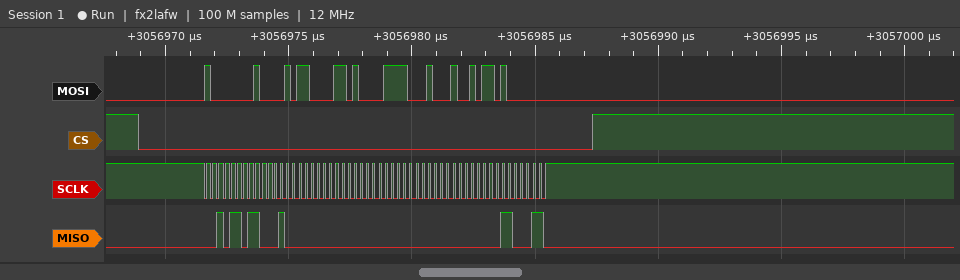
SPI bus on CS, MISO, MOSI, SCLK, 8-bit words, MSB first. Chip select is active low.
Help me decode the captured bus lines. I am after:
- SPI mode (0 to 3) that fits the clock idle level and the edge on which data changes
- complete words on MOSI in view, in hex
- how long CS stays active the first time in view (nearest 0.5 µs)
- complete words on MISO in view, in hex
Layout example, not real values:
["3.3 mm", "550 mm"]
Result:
["3", "80, 85, 86, 87, 88, 96, 80", "18.5 µs", "2D, 88, 00, 00, 00, 00, C6"]
